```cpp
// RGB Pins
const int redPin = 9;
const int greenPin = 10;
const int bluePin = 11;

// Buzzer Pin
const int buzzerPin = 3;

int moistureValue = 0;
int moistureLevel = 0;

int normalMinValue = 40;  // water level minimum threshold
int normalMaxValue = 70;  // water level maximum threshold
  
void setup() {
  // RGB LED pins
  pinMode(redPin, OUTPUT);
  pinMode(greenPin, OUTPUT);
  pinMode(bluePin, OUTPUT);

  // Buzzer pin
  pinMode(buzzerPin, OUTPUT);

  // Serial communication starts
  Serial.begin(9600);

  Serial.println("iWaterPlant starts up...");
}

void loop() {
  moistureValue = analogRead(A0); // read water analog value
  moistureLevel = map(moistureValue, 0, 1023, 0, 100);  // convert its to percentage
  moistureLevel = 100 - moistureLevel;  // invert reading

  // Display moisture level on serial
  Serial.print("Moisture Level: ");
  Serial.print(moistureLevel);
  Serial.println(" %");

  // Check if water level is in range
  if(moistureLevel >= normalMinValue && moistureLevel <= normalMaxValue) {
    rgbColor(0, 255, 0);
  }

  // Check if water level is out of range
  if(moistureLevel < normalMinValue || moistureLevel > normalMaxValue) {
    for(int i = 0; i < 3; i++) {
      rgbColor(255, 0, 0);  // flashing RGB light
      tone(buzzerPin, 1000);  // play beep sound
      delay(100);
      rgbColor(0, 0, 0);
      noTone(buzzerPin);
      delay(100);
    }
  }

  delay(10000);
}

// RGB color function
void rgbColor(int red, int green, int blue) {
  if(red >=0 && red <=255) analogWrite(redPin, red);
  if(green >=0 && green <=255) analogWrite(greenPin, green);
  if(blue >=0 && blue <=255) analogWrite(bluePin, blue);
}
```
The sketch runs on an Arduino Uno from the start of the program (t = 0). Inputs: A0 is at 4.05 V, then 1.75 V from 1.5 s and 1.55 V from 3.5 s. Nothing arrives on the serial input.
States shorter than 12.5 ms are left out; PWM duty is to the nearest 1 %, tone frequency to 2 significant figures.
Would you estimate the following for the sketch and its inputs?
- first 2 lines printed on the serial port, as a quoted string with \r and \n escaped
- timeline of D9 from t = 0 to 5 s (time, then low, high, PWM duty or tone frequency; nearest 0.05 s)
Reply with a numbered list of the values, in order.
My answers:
1. "iWaterPlant starts up...\r\nMoisture Level: 19 %\r\n"
2. 0 s high; 0.1 s low; 0.2 s high; 0.3 s low; 0.4 s high; 0.5 s low
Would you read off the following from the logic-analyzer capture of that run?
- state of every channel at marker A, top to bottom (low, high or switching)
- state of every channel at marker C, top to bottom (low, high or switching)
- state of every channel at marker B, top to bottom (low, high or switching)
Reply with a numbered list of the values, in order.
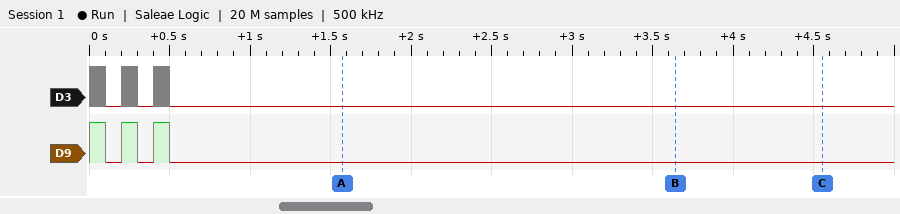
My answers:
1. D3 low, D9 low
2. D3 low, D9 low
3. D3 low, D9 low
